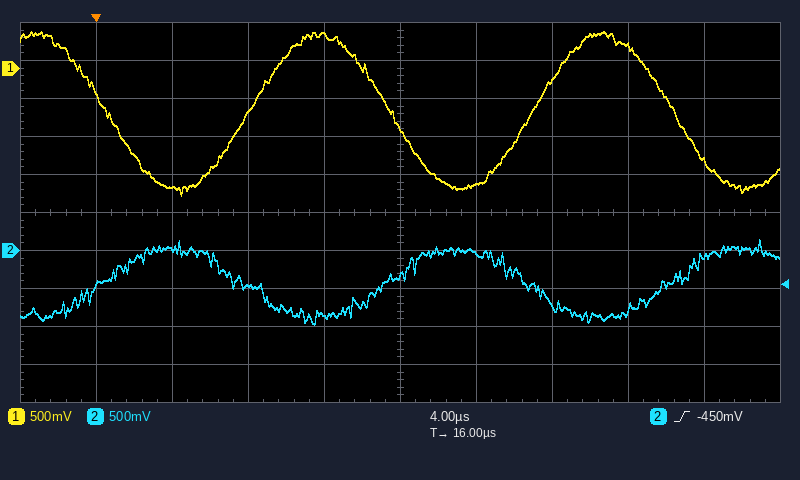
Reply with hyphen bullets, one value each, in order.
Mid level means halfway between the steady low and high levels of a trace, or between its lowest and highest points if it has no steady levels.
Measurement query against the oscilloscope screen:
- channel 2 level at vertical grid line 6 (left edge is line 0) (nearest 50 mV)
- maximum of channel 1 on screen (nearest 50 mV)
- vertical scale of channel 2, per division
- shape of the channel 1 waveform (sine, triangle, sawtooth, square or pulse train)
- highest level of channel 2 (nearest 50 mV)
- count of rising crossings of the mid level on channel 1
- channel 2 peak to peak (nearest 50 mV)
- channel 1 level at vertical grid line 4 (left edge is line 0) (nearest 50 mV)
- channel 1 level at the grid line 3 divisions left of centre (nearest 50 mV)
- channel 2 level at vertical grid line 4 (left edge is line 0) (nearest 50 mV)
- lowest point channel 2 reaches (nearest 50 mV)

- -50 mV
- 500 mV
- 500 mV
- sine
- 150 mV
- 2
- 1.10 V
- 450 mV
- -1.55 V
- -850 mV
- -950 mV
